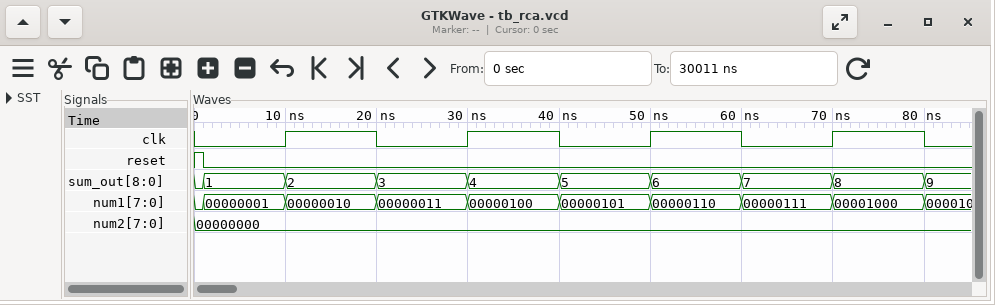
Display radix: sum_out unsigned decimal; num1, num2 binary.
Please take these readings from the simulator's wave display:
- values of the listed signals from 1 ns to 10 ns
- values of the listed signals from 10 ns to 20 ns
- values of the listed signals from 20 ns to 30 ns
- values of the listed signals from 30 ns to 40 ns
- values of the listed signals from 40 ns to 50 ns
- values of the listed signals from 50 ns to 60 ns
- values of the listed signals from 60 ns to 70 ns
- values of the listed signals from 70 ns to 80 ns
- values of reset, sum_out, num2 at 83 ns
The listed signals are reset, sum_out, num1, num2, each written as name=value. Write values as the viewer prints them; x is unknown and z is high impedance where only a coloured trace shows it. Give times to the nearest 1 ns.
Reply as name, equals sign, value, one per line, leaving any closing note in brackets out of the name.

values of the listed signals from 1 ns to 10 ns = reset=0, sum_out=1, num1=00000001, num2=00000000
values of the listed signals from 10 ns to 20 ns = reset=0, sum_out=2, num1=00000010, num2=00000000
values of the listed signals from 20 ns to 30 ns = reset=0, sum_out=3, num1=00000011, num2=00000000
values of the listed signals from 30 ns to 40 ns = reset=0, sum_out=4, num1=00000100, num2=00000000
values of the listed signals from 40 ns to 50 ns = reset=0, sum_out=5, num1=00000101, num2=00000000
values of the listed signals from 50 ns to 60 ns = reset=0, sum_out=6, num1=00000110, num2=00000000
values of the listed signals from 60 ns to 70 ns = reset=0, sum_out=7, num1=00000111, num2=00000000
values of the listed signals from 70 ns to 80 ns = reset=0, sum_out=8, num1=00001000, num2=00000000
values of reset, sum_out, num2 at 83 ns = reset=0, sum_out=9, num2=00000000
